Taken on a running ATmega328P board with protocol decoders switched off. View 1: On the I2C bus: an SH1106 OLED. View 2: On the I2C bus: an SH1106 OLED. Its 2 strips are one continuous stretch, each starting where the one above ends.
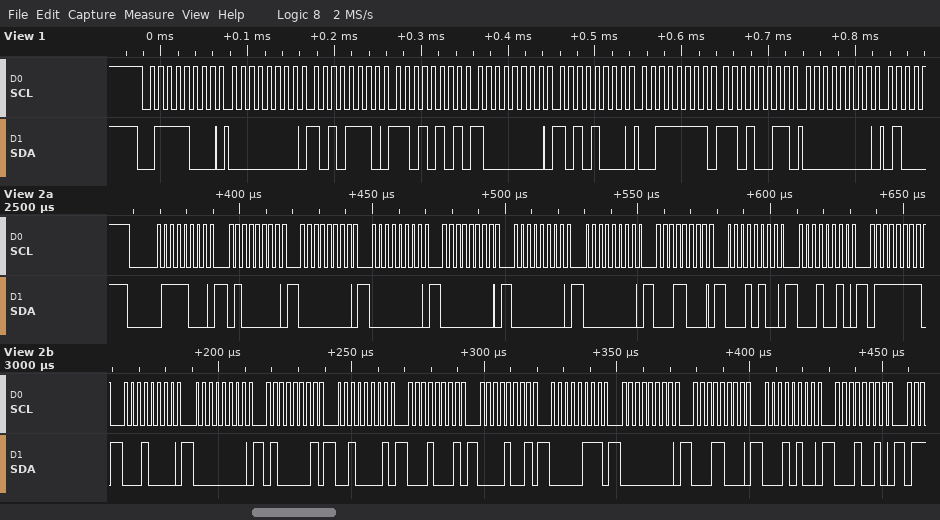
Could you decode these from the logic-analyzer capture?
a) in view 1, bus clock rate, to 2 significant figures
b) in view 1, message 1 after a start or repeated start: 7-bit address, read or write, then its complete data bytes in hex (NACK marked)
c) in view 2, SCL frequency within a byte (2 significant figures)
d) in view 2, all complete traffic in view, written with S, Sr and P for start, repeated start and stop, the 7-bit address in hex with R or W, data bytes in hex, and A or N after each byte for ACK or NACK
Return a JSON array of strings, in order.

["100 kHz", "0x3C write: 00 AE D5 80 A8 3F D3 00", "400 kHz", "S 3CW A 40 A 00 A 00 A 00 A 00 A 00 A 18 A 14 A 12 A 7F A 10 A 00 A 41 A 21 A 11 A 09 A 07 A 00 A 18 A 14 A 12 A"]
